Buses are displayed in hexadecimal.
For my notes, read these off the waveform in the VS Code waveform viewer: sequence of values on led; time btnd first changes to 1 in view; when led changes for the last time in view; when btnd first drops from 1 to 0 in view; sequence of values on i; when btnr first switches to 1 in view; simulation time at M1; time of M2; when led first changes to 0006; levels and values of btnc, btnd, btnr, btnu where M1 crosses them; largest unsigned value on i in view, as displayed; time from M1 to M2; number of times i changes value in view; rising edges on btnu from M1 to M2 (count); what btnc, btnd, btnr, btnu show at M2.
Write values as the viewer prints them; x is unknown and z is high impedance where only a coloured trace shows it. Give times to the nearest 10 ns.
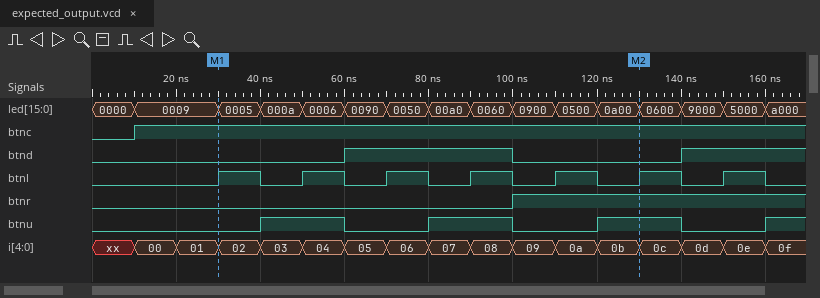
0000, 0009, 0005, 000a, 0006, 0090, 0050, 00a0, 0060, 0900, 0500, 0a00, 0600, 9000, 5000, a000
60 ns
160 ns
100 ns
xx, 00, 01, 02, 03, 04, 05, 06, 07, 08, 09, 0a, 0b, 0c, 0d, 0e, 0f
100 ns
30 ns
130 ns
50 ns
btnc=1, btnd=0, btnr=0, btnu=0
0f
100 ns
16
3
btnc=1, btnd=0, btnr=1, btnu=1
